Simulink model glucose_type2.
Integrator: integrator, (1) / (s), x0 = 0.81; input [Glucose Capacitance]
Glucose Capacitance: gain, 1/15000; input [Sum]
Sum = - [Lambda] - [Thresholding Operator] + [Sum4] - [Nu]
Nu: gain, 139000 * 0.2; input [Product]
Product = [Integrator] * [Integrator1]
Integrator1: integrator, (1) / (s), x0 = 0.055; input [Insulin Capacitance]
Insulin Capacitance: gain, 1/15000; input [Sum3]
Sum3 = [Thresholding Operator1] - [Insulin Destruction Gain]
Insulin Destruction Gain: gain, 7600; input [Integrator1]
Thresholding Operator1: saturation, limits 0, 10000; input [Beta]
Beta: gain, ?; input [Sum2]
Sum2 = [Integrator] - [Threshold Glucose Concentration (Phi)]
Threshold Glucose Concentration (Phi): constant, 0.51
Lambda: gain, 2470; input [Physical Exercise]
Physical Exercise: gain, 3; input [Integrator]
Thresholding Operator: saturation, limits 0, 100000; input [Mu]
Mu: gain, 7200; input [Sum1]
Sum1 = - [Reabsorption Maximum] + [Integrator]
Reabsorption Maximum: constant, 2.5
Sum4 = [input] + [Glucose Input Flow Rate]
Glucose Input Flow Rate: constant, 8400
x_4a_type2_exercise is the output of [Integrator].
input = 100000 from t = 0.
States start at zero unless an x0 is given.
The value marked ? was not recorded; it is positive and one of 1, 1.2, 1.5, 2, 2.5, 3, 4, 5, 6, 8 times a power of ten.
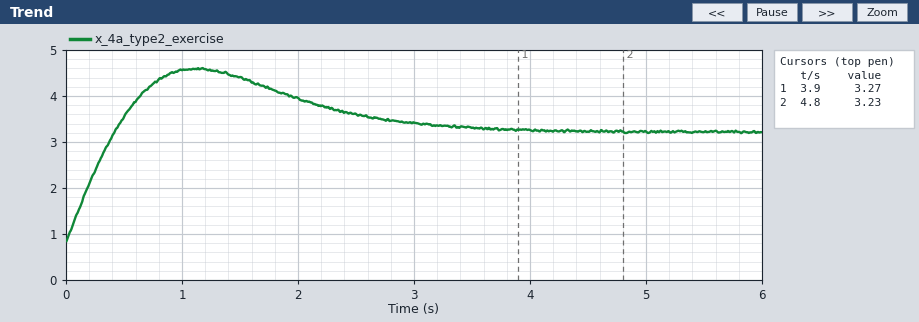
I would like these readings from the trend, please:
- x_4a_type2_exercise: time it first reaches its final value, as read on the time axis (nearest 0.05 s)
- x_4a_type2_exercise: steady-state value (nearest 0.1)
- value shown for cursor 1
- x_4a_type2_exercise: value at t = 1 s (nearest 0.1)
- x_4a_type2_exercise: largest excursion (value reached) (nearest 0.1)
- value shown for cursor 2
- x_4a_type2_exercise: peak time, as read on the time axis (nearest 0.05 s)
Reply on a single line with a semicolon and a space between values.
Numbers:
0.40 s; 3.2; 3.27; 4.6; 4.6; 3.23; 1.10 s
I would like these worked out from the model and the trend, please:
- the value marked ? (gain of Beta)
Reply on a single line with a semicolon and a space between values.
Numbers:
2500
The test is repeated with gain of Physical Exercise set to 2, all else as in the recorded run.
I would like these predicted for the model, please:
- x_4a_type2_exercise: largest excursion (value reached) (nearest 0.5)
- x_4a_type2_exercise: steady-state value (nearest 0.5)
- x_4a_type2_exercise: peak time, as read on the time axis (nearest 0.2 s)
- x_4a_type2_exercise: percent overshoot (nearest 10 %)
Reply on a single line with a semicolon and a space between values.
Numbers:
5.0; 3.5; 1.2 s; 60 %
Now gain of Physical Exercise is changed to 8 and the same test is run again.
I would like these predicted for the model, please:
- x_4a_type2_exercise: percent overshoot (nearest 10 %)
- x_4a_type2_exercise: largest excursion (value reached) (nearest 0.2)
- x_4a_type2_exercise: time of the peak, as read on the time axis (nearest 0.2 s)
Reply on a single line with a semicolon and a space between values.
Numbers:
40 %; 3.4; 1.0 s
